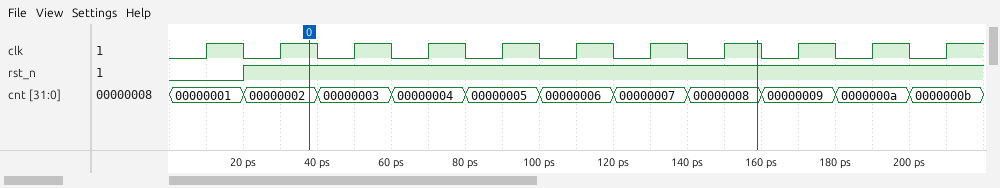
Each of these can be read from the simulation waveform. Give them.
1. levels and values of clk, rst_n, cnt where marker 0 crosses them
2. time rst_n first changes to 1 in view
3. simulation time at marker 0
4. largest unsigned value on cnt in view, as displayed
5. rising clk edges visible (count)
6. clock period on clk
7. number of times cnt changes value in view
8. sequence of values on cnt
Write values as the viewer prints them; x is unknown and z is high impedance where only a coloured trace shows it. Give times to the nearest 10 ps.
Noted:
clk=1, rst_n=1, cnt=00000002
20 ps
40 ps
0000000b
11
20 ps
10
00000001, 00000002, 00000003, 00000004, 00000005, 00000006, 00000007, 00000008, 00000009, 0000000a, 0000000b
